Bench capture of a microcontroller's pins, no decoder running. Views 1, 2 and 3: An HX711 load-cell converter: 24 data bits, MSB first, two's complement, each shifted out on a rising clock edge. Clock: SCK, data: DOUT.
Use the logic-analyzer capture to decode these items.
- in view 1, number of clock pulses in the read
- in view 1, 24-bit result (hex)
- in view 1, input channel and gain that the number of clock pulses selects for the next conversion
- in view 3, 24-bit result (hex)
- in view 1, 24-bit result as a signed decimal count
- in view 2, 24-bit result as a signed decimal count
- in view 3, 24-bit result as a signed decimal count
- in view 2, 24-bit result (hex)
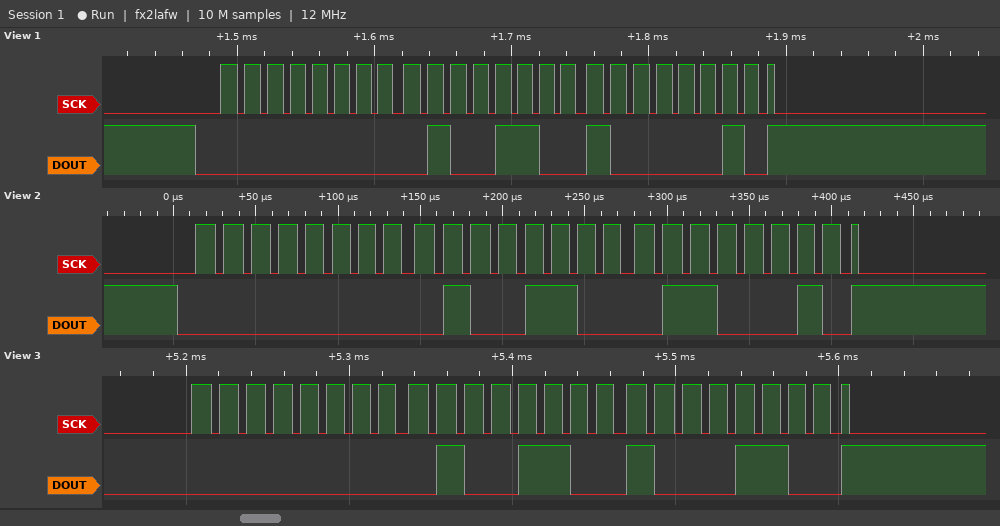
25
0x004C82
channel A, gain 128
0x004C8C
19586
19554
19596
0x004C62
